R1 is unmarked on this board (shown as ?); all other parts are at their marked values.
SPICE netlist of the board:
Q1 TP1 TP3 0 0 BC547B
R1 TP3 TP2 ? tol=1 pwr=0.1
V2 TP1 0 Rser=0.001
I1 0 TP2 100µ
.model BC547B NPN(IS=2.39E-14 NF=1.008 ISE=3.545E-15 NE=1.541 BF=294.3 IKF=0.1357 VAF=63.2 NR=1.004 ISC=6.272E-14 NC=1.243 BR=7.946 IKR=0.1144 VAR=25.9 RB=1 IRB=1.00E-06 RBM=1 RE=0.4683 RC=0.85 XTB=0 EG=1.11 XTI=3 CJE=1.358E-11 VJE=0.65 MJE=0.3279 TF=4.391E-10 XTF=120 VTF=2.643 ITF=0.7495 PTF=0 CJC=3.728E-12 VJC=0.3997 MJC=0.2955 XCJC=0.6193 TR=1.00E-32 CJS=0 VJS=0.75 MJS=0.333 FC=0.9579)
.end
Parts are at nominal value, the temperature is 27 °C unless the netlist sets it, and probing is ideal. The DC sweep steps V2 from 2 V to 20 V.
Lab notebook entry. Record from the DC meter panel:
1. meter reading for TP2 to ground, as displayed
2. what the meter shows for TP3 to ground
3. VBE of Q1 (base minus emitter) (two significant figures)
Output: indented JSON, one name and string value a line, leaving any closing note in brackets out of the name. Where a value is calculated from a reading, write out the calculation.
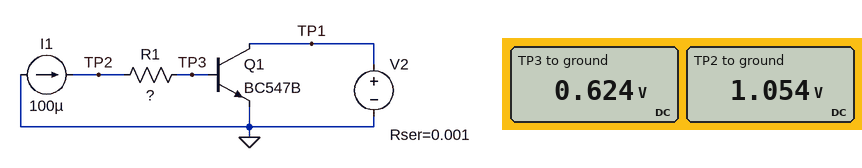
{
  "meter reading for TP2 to ground, as displayed": "1.054 V",
  "what the meter shows for TP3 to ground": "0.624 V",
  "VBE of Q1 (base minus emitter)": "624 mV = 620 mV"
}
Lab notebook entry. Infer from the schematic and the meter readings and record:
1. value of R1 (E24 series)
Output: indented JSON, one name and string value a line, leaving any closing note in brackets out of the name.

{
  "value of R1": "4.3 kΩ"
}
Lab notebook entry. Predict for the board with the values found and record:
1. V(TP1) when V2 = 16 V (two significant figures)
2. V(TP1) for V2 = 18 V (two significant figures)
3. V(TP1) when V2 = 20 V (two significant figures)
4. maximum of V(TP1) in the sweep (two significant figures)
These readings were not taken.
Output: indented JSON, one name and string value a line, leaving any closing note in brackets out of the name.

{
  "V(TP1) when V2 = 16 V": "16 V",
  "V(TP1) for V2 = 18 V": "18 V",
  "V(TP1) when V2 = 20 V": "20 V",
  "maximum of V(TP1) in the sweep": "20 V"
}
